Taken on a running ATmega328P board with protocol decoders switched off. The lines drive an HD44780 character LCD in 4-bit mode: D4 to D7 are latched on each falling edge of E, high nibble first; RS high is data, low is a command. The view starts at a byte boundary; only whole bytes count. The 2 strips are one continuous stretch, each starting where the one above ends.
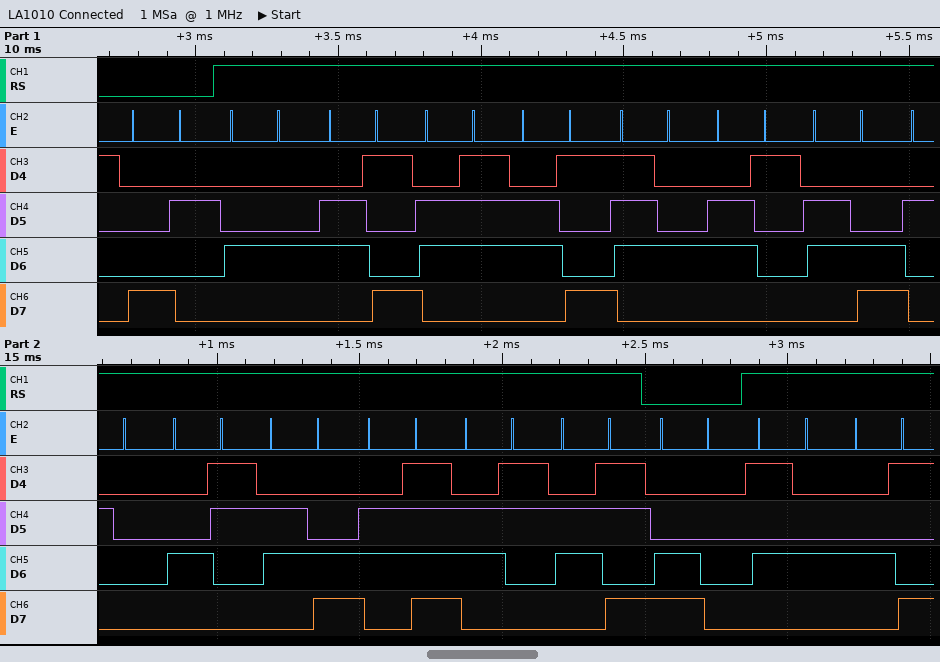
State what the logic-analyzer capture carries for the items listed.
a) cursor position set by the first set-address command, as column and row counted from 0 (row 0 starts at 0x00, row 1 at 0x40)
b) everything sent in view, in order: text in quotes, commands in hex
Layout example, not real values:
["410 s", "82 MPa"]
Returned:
["column 2, row 0", "0x82 \"Digital Clock\" 0xC0 \"TI\""]
